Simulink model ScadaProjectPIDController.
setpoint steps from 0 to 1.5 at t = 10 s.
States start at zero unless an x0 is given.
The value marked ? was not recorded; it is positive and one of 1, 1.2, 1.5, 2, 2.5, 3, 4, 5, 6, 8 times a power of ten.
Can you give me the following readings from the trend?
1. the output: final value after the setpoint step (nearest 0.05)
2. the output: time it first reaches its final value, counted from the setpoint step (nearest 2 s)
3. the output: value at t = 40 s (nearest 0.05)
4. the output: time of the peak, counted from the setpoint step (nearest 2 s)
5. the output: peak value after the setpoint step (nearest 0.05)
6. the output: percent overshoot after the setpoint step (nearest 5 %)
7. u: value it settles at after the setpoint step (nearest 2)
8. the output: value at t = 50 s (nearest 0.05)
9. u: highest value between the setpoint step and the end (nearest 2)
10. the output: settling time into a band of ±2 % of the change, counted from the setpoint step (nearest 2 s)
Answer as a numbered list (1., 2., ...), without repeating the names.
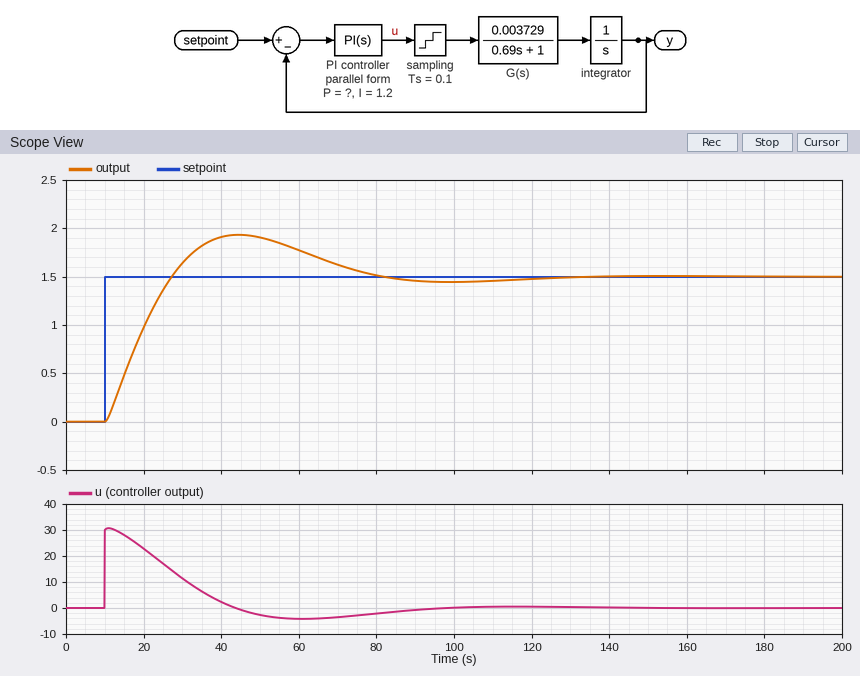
1. 1.50
2. 18 s
3. 1.90
4. 34 s
5. 1.95
6. 30 %
7. 0
8. 1.90
9. 30
10. 108 s
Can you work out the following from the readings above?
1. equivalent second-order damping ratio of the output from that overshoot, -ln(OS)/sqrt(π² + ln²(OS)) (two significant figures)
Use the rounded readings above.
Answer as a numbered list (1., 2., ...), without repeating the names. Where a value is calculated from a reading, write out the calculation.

1. ln(0.3) = -1.204; 1.204 / sqrt(9.870 + 1.450) = 0.36
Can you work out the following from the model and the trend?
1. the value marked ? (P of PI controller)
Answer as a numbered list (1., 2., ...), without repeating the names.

1. 20
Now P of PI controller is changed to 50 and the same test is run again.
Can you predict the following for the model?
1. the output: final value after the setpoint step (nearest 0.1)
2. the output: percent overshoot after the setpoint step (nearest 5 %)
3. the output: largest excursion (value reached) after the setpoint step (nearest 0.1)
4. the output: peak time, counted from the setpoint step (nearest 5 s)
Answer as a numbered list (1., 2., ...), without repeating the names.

1. 1.5
2. 10 %
3. 1.6
4. 25 s
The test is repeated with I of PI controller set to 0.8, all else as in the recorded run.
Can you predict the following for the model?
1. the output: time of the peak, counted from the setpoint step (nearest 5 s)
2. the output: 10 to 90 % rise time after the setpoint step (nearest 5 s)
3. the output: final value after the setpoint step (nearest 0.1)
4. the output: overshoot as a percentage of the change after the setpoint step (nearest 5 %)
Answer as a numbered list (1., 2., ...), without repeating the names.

1. 40 s
2. 15 s
3. 1.5
4. 25 %
